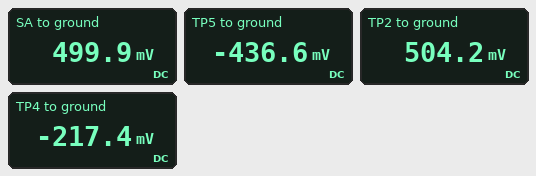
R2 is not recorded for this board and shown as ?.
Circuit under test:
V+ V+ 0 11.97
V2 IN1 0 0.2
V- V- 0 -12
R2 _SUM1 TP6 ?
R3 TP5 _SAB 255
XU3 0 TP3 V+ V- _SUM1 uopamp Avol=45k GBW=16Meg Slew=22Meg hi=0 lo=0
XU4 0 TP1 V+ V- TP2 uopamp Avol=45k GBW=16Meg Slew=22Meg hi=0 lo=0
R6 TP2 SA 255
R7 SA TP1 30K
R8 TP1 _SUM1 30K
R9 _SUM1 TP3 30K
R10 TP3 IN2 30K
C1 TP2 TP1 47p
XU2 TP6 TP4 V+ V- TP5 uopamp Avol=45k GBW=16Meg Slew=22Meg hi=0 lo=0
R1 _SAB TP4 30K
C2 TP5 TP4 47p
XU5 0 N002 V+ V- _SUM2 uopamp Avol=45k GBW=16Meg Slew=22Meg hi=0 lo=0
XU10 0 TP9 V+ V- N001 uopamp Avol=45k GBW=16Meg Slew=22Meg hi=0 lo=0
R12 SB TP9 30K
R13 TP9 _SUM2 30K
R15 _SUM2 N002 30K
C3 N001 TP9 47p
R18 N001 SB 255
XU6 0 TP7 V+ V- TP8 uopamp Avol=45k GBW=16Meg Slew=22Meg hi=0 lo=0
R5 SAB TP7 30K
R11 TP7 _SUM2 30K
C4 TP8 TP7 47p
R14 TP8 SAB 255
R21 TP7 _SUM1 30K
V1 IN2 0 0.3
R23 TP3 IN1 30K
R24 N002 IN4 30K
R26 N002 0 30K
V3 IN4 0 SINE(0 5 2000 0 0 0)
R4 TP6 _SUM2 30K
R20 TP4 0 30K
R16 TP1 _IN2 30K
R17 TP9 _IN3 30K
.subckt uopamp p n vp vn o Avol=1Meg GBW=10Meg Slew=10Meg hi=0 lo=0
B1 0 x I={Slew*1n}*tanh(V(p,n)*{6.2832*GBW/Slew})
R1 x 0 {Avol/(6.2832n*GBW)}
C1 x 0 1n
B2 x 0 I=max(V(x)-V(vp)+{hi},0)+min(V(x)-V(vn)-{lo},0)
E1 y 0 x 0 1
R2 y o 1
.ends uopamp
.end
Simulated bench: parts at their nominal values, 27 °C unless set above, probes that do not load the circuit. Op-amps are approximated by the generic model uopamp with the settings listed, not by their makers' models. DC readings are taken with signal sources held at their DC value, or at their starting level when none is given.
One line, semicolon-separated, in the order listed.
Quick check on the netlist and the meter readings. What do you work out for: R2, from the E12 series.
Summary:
39 kΩ
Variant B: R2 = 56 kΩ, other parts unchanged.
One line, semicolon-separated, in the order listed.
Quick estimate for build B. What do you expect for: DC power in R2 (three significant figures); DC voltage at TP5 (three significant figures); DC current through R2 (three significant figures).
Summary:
1.89 µW; -350 mV; 5.81 µA
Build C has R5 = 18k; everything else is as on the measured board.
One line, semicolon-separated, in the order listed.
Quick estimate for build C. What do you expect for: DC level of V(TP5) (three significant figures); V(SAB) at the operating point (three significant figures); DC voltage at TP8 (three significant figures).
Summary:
-437 mV; 300 mV; 304 mV
